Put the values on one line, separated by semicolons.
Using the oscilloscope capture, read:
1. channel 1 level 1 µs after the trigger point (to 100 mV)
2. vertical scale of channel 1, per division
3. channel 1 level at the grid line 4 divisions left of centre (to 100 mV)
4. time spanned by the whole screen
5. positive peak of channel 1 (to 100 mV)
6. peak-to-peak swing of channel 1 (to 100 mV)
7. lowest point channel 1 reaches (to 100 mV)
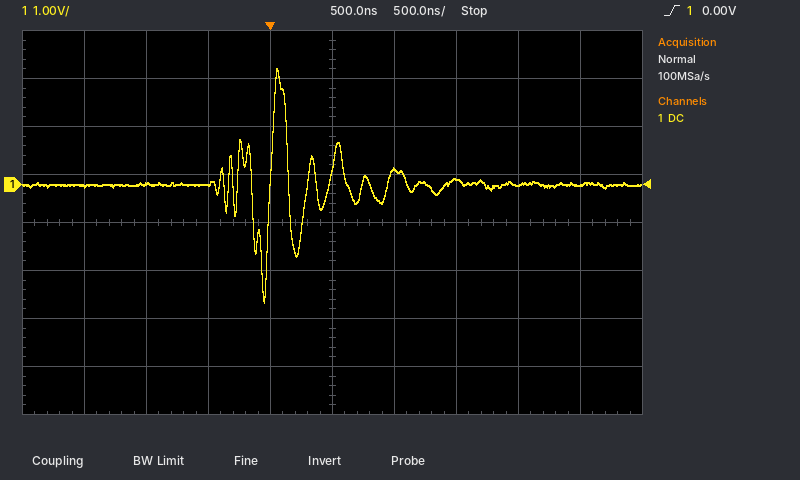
300 mV; 1 V; 0.0 V; 5 µs; 2.4 V; 4.9 V; -2.5 V
